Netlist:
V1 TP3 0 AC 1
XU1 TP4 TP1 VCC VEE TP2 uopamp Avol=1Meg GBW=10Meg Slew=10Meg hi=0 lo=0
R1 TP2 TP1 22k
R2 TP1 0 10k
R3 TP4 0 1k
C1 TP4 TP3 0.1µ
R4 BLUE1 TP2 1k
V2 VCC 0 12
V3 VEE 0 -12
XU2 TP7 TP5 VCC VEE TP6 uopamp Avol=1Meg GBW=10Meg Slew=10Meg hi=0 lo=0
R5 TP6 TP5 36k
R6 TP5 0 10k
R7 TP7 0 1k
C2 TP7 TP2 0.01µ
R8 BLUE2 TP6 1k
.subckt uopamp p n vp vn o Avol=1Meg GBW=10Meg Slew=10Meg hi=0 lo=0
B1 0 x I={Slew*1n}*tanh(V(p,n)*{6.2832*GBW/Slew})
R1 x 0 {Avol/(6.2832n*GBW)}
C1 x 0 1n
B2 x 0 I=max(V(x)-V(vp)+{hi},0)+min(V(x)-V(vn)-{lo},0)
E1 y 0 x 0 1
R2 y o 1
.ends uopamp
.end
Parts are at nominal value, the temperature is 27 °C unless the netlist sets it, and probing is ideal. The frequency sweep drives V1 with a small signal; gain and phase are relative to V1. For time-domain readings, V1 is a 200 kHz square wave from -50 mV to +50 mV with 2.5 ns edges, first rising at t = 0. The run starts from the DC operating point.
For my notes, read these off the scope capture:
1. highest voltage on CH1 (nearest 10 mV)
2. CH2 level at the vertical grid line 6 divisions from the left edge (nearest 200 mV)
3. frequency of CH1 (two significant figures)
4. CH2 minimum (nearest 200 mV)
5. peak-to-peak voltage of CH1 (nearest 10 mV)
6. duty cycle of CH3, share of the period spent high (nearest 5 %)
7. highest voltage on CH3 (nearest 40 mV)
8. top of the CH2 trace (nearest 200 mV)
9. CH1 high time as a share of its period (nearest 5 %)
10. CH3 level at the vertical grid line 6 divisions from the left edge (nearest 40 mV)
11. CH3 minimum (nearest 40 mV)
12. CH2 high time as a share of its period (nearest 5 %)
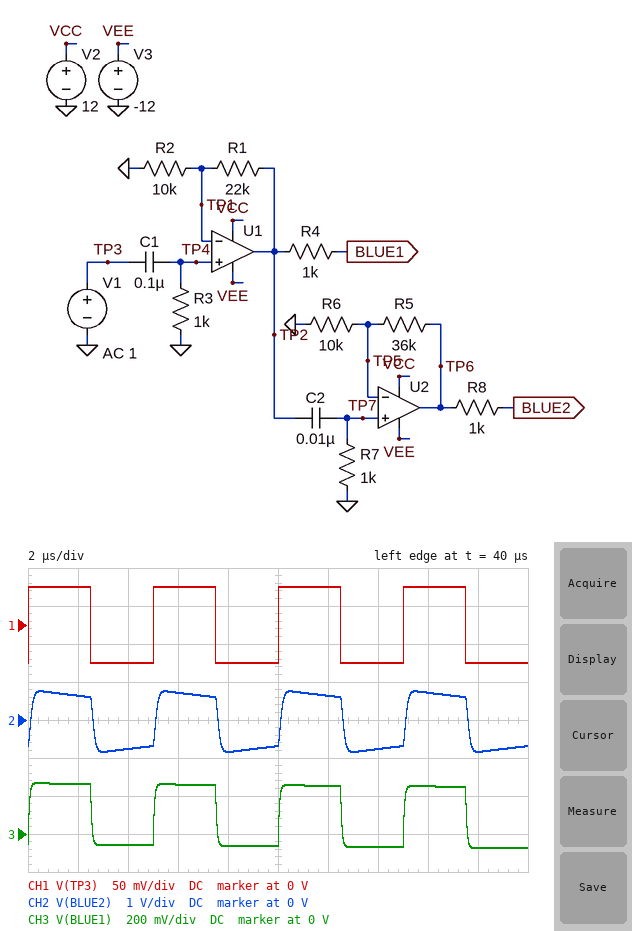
50 mV
600 mV
200 kHz
-800 mV
100 mV
50 %
280 mV
800 mV
50 %
240 mV
-80 mV
50 %
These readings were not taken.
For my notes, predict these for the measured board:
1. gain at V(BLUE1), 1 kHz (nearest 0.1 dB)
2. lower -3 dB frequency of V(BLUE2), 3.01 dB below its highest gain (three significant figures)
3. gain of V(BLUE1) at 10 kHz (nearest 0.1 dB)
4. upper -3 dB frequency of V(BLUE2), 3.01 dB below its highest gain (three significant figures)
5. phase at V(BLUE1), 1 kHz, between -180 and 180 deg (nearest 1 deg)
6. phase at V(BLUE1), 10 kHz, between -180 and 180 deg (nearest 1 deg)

4.6 dB
15.8 kHz
10.0 dB
1.66 MHz
58 deg
9 deg
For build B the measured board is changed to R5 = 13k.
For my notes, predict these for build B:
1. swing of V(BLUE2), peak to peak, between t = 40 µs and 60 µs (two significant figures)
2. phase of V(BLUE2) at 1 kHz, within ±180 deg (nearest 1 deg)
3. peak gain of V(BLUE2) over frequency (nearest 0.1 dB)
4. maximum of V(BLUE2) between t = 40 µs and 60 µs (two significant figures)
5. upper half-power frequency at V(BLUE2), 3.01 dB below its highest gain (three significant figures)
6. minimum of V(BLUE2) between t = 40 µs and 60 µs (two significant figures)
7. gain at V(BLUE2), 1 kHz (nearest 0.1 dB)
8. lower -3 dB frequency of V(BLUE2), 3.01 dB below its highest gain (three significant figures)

810 mV
144 deg
17.3 dB
380 mV
2.35 MHz
-430 mV
-12.2 dB
15.9 kHz
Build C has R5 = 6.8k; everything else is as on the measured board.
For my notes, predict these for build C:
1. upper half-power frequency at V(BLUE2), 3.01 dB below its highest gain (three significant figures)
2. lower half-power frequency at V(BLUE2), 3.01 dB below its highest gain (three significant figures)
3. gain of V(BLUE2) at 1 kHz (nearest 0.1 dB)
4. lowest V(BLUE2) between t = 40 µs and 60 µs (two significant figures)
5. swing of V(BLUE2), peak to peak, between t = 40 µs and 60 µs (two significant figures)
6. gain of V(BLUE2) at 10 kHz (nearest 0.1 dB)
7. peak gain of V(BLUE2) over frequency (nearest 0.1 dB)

2.61 MHz
15.9 kHz
-14.9 dB
-310 mV
590 mV
9.0 dB
14.6 dB
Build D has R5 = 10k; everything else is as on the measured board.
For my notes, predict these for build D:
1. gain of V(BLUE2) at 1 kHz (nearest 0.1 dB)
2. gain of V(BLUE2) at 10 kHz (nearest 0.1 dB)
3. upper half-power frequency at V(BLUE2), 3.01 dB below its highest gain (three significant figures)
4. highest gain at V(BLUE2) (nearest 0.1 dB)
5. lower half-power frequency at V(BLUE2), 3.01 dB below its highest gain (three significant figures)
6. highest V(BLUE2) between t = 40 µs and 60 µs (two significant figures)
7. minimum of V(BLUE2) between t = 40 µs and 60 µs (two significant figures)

-13.4 dB
10.5 dB
2.47 MHz
16.1 dB
15.9 kHz
330 mV
-370 mV
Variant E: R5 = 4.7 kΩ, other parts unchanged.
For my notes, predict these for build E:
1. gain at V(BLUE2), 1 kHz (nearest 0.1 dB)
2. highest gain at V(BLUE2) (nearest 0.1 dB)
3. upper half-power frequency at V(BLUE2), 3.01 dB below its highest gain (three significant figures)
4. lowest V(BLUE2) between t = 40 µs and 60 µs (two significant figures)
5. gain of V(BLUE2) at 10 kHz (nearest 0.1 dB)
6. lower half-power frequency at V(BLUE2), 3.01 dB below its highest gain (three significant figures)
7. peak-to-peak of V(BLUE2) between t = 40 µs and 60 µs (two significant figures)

-16.1 dB
13.4 dB
2.70 MHz
-270 mV
7.9 dB
15.9 kHz
520 mV
